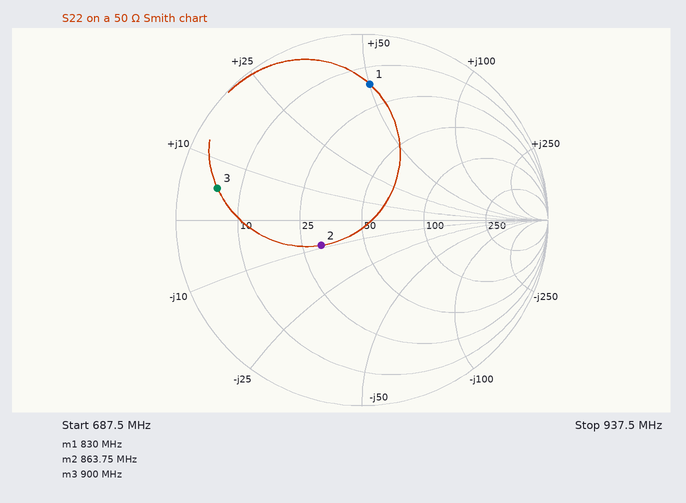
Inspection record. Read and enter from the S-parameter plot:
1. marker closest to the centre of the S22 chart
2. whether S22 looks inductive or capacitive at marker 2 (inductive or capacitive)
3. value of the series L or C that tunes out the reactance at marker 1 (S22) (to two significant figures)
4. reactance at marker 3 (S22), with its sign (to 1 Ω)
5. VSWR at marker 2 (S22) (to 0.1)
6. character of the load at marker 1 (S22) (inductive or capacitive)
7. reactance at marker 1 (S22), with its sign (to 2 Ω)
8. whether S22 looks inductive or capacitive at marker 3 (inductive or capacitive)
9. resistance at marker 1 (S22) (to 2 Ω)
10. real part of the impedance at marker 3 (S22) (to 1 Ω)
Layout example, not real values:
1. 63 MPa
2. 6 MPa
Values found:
1. marker 2
2. capacitive
3. 3.8 pF
4. +5 Ω
5. 1.7
6. inductive
7. +50 Ω
8. inductive
9. 16 Ω
10. 6 Ω
